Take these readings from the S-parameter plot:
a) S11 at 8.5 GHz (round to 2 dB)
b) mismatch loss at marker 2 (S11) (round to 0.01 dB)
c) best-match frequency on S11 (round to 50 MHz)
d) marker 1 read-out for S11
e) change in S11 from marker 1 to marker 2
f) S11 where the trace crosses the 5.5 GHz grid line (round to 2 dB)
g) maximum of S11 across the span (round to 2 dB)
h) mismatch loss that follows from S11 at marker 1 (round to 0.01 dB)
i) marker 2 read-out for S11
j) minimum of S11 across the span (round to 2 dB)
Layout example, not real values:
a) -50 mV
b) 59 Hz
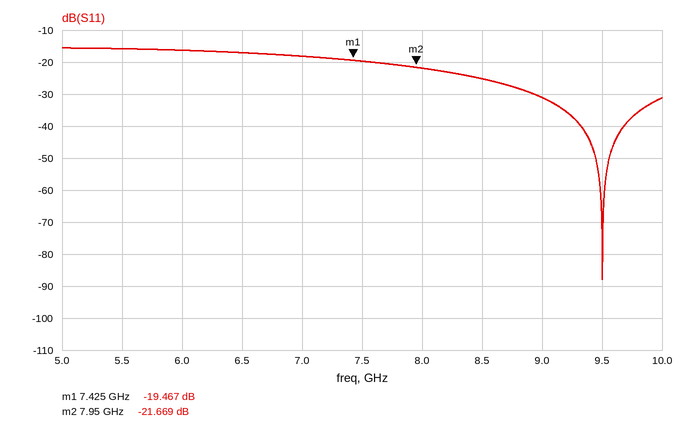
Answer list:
a) -26 dB
b) 0.03 dB
c) 9.50 GHz
d) -19.467 dB
e) -2.202 dB
f) -16 dB
g) -16 dB
h) 0.05 dB
i) -21.669 dB
j) -88 dB
